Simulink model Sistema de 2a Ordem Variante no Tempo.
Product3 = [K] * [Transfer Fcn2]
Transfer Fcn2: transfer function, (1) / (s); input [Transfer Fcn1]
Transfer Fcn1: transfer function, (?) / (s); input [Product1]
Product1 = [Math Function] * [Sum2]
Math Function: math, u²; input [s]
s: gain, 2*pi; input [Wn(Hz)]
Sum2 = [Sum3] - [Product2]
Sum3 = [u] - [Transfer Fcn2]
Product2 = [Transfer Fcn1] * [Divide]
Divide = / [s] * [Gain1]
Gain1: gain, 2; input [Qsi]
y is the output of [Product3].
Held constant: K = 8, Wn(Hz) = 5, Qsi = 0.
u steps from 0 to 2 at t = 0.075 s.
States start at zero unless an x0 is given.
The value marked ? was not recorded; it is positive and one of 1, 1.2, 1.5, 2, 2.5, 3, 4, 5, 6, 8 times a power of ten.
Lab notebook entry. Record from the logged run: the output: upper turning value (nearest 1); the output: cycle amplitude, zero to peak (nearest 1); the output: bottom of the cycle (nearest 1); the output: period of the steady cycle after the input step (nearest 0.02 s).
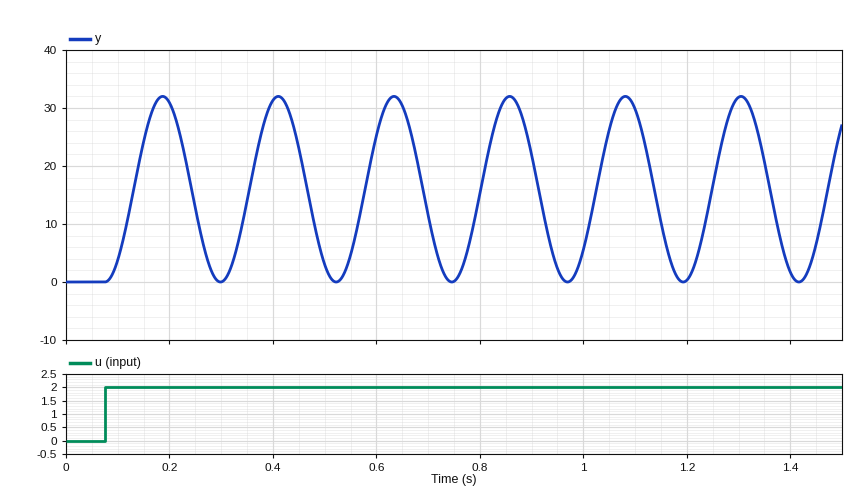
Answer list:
32
16
0
0.22 s
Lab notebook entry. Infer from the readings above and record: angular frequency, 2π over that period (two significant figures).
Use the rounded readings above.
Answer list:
29 rad/s
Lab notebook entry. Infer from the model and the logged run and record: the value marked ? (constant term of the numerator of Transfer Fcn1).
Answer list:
0.8
